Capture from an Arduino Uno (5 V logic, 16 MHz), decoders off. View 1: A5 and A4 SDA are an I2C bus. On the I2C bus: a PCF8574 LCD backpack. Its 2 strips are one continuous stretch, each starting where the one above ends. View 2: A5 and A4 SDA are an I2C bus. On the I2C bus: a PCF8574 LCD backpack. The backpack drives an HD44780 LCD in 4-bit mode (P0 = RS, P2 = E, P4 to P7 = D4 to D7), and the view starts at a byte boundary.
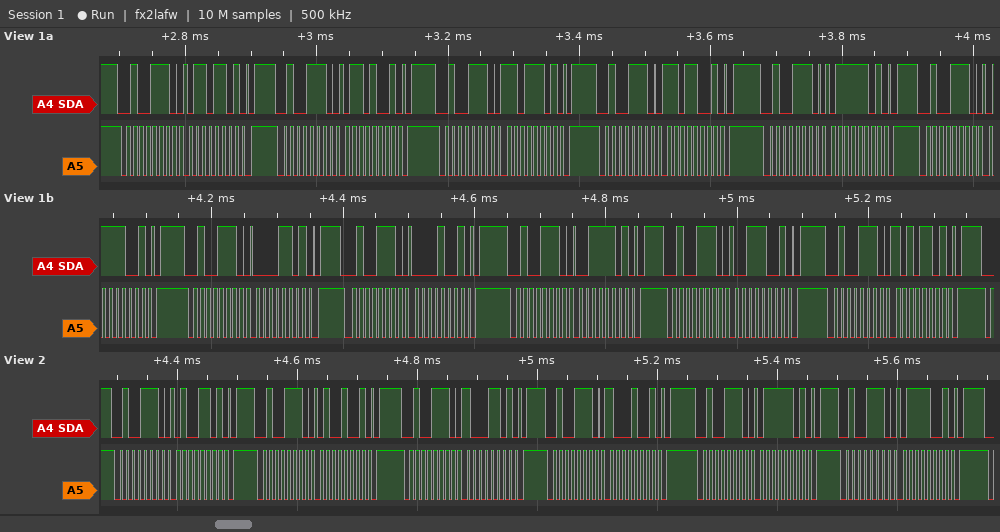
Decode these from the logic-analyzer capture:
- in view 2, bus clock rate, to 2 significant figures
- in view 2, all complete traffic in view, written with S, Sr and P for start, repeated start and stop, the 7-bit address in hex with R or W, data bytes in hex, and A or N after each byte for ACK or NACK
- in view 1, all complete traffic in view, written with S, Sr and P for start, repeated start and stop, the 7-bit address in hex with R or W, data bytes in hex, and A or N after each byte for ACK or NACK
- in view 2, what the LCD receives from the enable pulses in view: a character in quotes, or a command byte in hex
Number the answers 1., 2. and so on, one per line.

1. 100 kHz
2. S 27W A 4D A P S 27W A 49 A P S 27W A 8D A P S 27W A 89 A P S 27W A 7D A P S 27W A 79 A P
3. S 27W A 6D A P S 27W A 69 A P S 27W A DD A P S 27W A D9 A P S 27W A 7D A P S 27W A 79 A P S 27W A 0D A P S 27W A 09 A P S 27W A 3D A P S 27W A 39 A P S 27W A AD A P
4. 'H'
